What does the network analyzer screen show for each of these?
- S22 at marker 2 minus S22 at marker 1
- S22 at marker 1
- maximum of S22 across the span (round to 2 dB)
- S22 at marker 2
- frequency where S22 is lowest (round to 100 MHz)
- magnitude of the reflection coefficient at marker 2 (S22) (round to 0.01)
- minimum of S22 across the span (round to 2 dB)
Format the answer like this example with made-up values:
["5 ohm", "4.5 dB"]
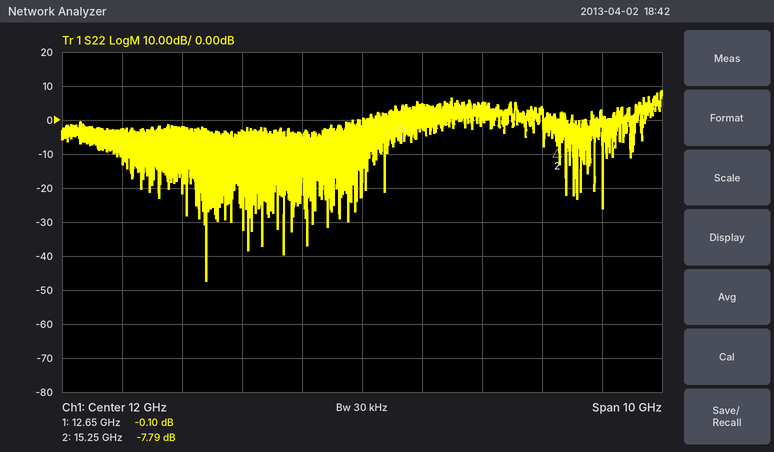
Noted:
["-7.69 dB", "-0.10 dB", "8 dB", "-7.79 dB", "9.4 GHz", "0.41", "-48 dB"]
